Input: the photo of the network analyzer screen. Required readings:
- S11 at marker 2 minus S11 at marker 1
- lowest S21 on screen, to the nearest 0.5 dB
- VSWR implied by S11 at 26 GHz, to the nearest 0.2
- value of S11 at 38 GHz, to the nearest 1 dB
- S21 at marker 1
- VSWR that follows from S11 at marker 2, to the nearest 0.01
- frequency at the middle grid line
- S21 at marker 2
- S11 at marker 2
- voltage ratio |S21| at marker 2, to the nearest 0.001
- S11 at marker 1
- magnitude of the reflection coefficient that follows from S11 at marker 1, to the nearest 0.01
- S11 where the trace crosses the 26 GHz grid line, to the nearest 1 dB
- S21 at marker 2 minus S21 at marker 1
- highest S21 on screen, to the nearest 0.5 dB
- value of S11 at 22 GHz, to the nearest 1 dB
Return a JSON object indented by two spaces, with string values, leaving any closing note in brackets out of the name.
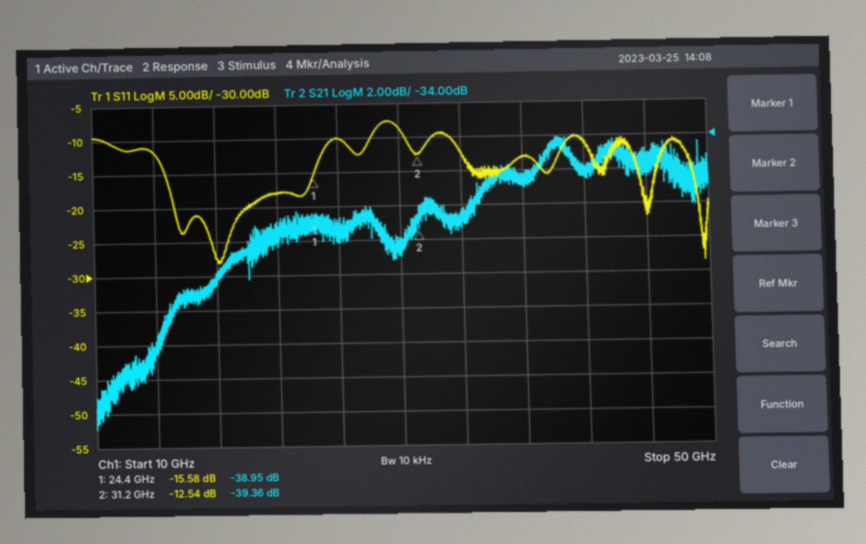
{
  "S11 at marker 2 minus S11 at marker 1": "3.04 dB",
  "lowest S21 on screen, to the nearest 0.5 dB": "-51.0 dB",
  "VSWR implied by S11 at 26 GHz, to the nearest 0.2": "2.0",
  "value of S11 at 38 GHz, to the nearest 1 dB": "-13 dB",
  "S21 at marker 1": "-38.95 dB",
  "VSWR that follows from S11 at marker 2, to the nearest 0.01": "1.62",
  "frequency at the middle grid line": "30 GHz",
  "S21 at marker 2": "-39.36 dB",
  "S11 at marker 2": "-12.54 dB",
  "voltage ratio |S21| at marker 2, to the nearest 0.001": "0.011",
  "S11 at marker 1": "-15.58 dB",
  "magnitude of the reflection coefficient that follows from S11 at marker 1, to the nearest 0.01": "0.17",
  "S11 where the trace crosses the 26 GHz grid line, to the nearest 1 dB": "-10 dB",
  "S21 at marker 2 minus S21 at marker 1": "-0.41 dB",
  "highest S21 on screen, to the nearest 0.5 dB": "-34.0 dB",
  "value of S11 at 22 GHz, to the nearest 1 dB": "-18 dB"
}
